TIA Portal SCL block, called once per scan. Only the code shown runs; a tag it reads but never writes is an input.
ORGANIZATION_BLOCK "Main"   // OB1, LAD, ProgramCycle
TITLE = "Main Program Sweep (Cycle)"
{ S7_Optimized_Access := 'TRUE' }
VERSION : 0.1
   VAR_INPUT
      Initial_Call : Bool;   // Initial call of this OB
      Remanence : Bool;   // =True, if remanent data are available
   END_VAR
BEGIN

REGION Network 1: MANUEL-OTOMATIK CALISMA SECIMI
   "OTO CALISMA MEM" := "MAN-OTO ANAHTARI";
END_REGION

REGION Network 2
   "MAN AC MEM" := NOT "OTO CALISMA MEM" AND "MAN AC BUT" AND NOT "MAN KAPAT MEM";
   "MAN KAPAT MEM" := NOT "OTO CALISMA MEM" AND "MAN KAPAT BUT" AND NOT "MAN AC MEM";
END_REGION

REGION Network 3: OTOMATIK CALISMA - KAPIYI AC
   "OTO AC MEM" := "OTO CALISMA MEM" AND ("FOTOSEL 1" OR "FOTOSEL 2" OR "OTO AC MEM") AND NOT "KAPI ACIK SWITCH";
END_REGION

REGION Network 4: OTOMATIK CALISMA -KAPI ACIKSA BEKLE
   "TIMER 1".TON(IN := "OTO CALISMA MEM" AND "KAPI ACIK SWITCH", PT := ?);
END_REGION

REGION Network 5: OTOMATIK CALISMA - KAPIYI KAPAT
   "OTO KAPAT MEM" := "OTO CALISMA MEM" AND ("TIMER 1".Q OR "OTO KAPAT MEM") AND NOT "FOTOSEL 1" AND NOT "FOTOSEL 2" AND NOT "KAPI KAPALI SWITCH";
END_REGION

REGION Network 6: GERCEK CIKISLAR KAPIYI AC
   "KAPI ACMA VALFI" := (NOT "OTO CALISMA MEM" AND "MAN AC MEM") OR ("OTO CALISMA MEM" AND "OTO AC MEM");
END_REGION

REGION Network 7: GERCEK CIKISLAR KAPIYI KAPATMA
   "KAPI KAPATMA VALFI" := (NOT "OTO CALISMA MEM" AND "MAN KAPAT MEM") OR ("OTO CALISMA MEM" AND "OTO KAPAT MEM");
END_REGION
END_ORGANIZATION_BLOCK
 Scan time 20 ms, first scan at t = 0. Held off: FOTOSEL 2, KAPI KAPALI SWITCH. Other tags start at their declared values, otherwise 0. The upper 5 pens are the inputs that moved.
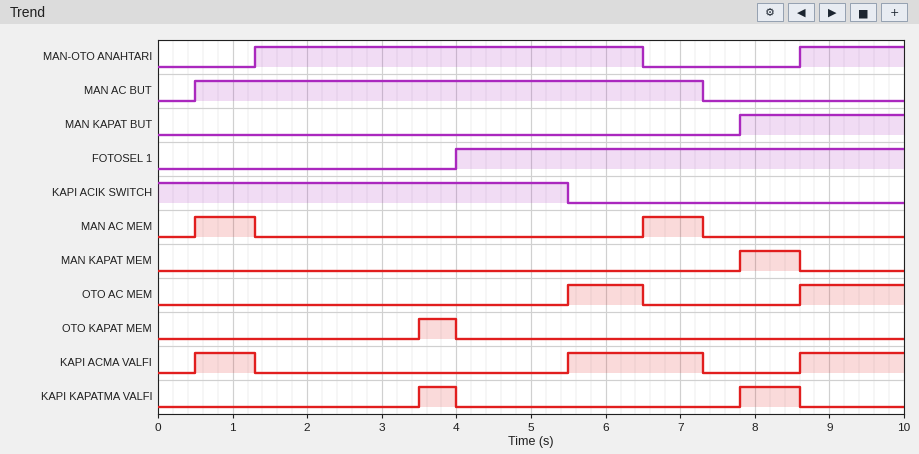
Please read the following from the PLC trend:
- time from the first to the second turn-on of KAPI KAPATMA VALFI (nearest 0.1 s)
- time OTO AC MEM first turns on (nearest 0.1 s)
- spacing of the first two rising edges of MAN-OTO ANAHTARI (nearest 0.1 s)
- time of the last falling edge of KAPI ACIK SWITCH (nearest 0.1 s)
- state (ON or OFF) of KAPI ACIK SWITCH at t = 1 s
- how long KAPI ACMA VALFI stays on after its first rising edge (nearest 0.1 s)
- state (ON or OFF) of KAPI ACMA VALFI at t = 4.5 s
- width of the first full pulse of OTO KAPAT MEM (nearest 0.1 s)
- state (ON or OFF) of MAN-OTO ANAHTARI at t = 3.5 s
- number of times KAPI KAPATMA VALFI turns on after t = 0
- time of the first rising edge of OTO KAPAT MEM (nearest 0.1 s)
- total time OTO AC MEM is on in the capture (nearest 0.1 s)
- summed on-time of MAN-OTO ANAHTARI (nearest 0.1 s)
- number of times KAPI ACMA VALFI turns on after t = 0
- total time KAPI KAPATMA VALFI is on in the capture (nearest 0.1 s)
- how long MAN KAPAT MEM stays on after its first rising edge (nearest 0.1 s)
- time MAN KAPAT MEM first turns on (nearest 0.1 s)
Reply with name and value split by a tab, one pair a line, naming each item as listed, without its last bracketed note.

time from the first to the second turn-on of KAPI KAPATMA VALFI	4.3 s
time OTO AC MEM first turns on	5.5 s
spacing of the first two rising edges of MAN-OTO ANAHTARI	7.3 s
time of the last falling edge of KAPI ACIK SWITCH	5.5 s
state (ON or OFF) of KAPI ACIK SWITCH at t = 1 s	ON
how long KAPI ACMA VALFI stays on after its first rising edge	0.8 s
state (ON or OFF) of KAPI ACMA VALFI at t = 4.5 s	OFF
width of the first full pulse of OTO KAPAT MEM	0.5 s
state (ON or OFF) of MAN-OTO ANAHTARI at t = 3.5 s	ON
number of times KAPI KAPATMA VALFI turns on after t = 0	2
time of the first rising edge of OTO KAPAT MEM	3.5 s
total time OTO AC MEM is on in the capture	2.4 s
summed on-time of MAN-OTO ANAHTARI	6.6 s
number of times KAPI ACMA VALFI turns on after t = 0	3
total time KAPI KAPATMA VALFI is on in the capture	1.3 s
how long MAN KAPAT MEM stays on after its first rising edge	0.8 s
time MAN KAPAT MEM first turns on	7.8 s
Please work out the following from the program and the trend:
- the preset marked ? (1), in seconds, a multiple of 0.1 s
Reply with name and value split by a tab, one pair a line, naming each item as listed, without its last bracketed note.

the preset marked ? (1), in seconds, a multiple of 0.1 s	2.2 s
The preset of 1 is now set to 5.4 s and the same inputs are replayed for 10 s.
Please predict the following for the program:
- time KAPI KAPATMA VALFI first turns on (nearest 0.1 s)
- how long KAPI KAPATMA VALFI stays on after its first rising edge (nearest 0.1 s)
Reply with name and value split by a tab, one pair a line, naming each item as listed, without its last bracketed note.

time KAPI KAPATMA VALFI first turns on	7.8 s
how long KAPI KAPATMA VALFI stays on after its first rising edge	0.8 s
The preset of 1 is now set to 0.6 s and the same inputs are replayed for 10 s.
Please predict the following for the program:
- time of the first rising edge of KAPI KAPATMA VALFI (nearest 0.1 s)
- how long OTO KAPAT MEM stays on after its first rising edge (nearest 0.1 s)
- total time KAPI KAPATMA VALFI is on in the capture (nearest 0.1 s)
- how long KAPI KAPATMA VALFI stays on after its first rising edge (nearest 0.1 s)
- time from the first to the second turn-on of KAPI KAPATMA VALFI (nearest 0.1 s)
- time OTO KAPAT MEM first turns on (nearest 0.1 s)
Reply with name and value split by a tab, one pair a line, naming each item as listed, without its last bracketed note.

time of the first rising edge of KAPI KAPATMA VALFI	1.9 s
how long OTO KAPAT MEM stays on after its first rising edge	2.1 s
total time KAPI KAPATMA VALFI is on in the capture	2.9 s
how long KAPI KAPATMA VALFI stays on after its first rising edge	2.1 s
time from the first to the second turn-on of KAPI KAPATMA VALFI	5.9 s
time OTO KAPAT MEM first turns on	1.9 s
